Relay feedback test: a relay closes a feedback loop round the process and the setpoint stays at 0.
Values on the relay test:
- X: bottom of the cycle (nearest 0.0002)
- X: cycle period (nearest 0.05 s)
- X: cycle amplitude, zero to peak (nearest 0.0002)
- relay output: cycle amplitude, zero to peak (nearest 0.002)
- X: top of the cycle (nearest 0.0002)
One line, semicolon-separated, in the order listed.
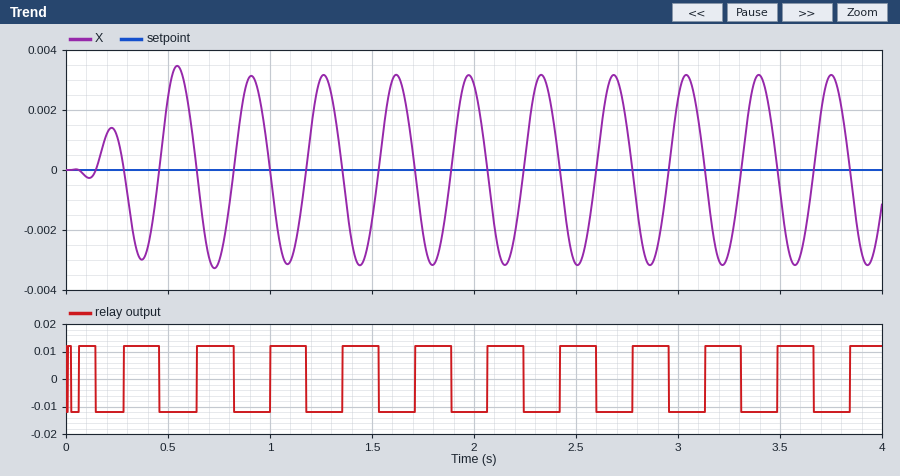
-0.0032; 0.35 s; 0.0032; 0.012; 0.0032
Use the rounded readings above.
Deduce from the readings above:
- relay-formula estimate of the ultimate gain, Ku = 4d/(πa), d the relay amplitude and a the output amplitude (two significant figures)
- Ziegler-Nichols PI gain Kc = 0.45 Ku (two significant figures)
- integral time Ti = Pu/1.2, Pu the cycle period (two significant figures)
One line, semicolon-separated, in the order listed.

4.8; 2.2; 0.29 s
